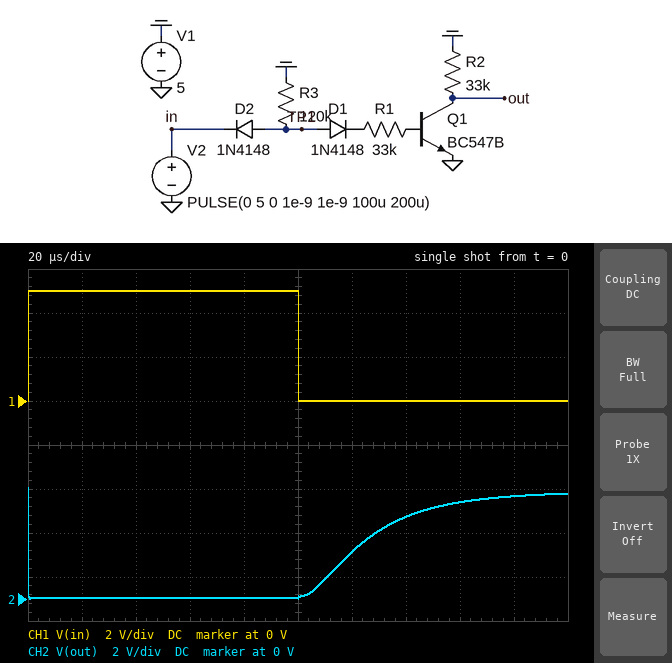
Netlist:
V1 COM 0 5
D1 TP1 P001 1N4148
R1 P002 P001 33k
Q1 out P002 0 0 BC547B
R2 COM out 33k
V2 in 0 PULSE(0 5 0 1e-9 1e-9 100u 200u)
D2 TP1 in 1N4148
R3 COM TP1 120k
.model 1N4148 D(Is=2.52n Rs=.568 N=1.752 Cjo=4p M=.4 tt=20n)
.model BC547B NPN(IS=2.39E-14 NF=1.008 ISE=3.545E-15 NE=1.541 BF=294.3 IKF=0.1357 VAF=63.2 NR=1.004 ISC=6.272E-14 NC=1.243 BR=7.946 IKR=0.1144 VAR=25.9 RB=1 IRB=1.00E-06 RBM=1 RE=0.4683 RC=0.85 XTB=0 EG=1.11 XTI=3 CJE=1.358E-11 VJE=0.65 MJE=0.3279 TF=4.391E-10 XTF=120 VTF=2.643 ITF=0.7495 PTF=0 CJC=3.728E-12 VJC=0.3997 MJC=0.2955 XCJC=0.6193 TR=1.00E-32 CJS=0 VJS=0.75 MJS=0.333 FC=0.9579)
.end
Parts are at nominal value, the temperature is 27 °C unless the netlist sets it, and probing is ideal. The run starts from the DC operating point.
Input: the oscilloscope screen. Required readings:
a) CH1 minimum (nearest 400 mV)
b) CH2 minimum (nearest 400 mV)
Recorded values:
0 V
0 V
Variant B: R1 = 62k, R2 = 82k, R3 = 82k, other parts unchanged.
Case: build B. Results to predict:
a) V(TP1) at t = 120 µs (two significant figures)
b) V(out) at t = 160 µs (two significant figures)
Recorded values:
450 mV
2.7 V
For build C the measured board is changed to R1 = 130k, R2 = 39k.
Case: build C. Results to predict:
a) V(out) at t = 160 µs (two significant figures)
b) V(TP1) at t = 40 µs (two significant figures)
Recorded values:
4.2 V
3.1 V
